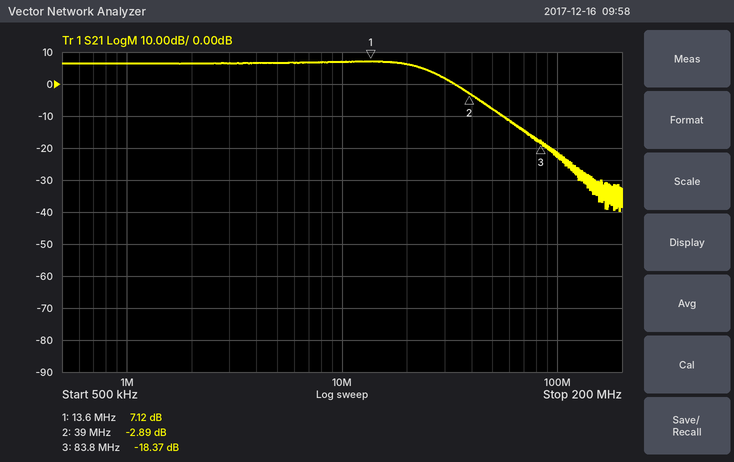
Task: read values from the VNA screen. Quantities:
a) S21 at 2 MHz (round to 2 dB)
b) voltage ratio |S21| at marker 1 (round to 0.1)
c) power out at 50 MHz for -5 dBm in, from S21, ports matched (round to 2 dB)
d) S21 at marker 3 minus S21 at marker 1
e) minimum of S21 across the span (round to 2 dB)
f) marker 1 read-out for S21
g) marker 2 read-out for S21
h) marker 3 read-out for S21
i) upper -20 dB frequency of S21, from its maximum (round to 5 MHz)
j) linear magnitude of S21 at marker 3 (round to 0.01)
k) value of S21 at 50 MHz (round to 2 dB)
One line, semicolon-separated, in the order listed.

6 dB; 2.3; -12 dBm; -25.49 dB; -40 dB; 7.12 dB; -2.89 dB; -18.37 dB; 65 MHz; 0.12; -8 dB
